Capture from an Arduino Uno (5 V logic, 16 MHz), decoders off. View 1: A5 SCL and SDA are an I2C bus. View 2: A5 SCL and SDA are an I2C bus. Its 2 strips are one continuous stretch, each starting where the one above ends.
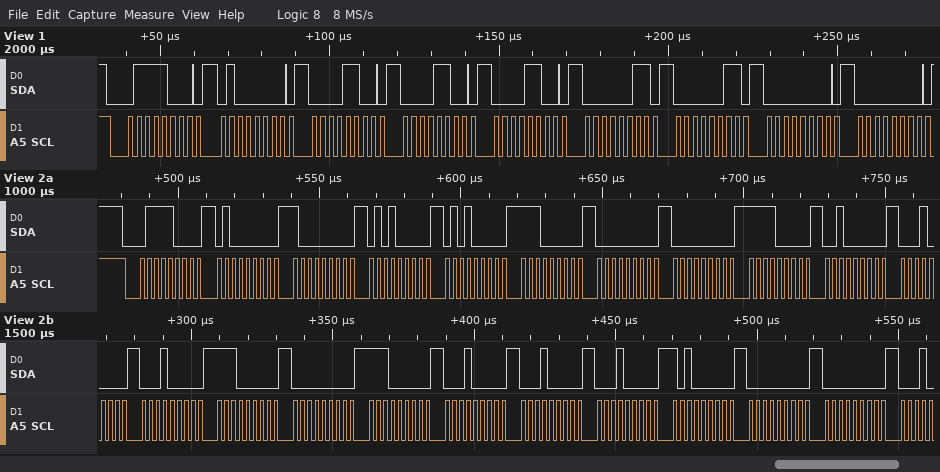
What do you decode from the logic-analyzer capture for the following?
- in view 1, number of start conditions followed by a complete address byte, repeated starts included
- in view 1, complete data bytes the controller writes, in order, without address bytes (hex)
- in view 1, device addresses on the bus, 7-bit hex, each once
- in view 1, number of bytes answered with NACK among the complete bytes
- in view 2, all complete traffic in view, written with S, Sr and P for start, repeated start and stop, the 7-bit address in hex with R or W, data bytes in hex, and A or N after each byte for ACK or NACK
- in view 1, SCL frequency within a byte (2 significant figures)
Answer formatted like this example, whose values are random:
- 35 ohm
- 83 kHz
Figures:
- 1
- 40 0C 0C 0C 03 03 00 00
- 0x3C
- 0
- S 3CW A 40 A 80 A 50 A 50 A E0 A 00 A 00 A F0 A 20 A 10 A 10 A E0 A 00 A E0 A 10 A 10 A 10 A A0 A 00 A 00 A
- 400 kHz
